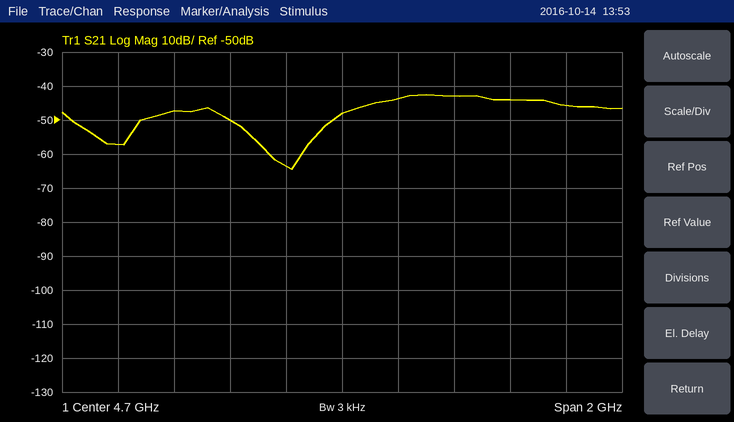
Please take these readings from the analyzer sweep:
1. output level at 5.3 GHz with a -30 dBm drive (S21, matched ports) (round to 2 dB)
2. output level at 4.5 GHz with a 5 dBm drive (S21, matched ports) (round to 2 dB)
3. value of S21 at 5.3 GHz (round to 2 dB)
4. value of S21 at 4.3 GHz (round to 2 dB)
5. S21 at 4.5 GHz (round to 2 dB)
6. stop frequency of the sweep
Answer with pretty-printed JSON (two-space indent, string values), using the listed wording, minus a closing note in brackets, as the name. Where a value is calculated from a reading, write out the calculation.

{
  "output level at 5.3 GHz with a -30 dBm drive (S21, matched ports)": "-30 dBm + (-44 dB) = -74 dBm",
  "output level at 4.5 GHz with a 5 dBm drive (S21, matched ports)": "5 dBm + (-64 dB) = -58 dBm",
  "value of S21 at 5.3 GHz": "-44 dB",
  "value of S21 at 4.3 GHz": "-50 dB",
  "S21 at 4.5 GHz": "-64 dB",
  "stop frequency of the sweep": "5.7 GHz"
}
